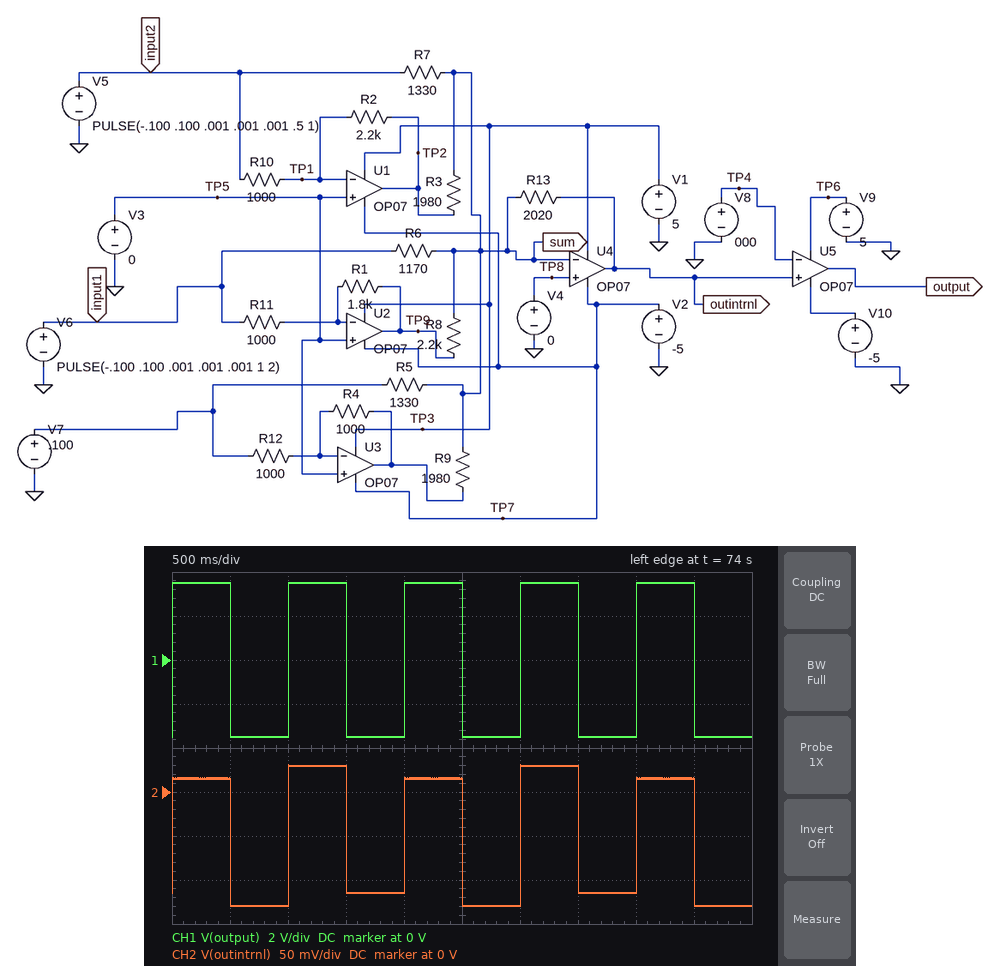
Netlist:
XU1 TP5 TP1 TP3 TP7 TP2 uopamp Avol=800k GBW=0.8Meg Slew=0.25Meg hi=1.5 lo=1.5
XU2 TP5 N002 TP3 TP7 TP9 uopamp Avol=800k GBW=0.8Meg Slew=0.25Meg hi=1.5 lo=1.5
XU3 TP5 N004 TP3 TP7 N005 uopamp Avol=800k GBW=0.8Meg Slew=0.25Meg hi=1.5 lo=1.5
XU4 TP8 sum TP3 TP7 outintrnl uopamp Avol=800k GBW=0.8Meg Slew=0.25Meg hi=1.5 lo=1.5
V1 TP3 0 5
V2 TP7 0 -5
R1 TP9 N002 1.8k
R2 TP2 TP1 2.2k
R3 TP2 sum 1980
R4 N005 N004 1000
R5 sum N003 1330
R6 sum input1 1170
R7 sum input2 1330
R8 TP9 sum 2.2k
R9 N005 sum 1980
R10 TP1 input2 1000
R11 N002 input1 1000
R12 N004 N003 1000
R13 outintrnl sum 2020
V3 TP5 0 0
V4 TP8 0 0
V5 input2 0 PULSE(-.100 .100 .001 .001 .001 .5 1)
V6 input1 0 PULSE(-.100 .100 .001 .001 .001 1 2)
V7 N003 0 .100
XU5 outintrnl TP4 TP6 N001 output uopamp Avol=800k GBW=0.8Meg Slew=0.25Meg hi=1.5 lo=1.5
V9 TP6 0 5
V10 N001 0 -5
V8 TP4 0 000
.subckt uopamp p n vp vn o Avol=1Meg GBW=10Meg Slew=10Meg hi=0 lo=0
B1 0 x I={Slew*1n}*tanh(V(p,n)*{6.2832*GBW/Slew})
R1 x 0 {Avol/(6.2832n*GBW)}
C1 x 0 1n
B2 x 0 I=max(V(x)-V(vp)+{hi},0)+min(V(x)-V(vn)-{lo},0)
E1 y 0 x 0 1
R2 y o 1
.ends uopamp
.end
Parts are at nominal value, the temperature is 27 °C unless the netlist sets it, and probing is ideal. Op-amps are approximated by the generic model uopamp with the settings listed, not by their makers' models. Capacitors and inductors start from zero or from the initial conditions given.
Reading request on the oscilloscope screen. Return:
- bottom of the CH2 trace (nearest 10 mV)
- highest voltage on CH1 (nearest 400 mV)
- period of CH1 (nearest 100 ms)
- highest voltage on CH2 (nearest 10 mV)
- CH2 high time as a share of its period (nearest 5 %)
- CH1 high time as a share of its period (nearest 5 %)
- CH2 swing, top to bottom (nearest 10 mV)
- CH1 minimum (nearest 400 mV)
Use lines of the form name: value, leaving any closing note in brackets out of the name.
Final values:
bottom of the CH2 trace: -130 mV
highest voltage on CH1: 3.6 V
period of CH1: 1.0 s
highest voltage on CH2: 30 mV
CH2 high time as a share of its period: 50 %
CH1 high time as a share of its period: 50 %
CH2 swing, top to bottom: 160 mV
CH1 minimum: -3.6 V
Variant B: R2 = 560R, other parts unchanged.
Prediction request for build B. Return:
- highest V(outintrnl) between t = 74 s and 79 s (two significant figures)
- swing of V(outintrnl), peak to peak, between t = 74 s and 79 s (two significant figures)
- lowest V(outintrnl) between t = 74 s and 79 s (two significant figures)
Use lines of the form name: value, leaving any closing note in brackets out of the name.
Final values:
highest V(outintrnl) between t = 74 s and 79 s: 52 mV
swing of V(outintrnl), peak to peak, between t = 74 s and 79 s: 200 mV
lowest V(outintrnl) between t = 74 s and 79 s: -150 mV
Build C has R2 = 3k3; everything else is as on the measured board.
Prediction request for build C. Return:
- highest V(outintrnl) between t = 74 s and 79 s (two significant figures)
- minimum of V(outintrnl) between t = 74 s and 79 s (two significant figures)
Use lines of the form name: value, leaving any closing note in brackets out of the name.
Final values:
highest V(outintrnl) between t = 74 s and 79 s: 140 mV
minimum of V(outintrnl) between t = 74 s and 79 s: -240 mV
